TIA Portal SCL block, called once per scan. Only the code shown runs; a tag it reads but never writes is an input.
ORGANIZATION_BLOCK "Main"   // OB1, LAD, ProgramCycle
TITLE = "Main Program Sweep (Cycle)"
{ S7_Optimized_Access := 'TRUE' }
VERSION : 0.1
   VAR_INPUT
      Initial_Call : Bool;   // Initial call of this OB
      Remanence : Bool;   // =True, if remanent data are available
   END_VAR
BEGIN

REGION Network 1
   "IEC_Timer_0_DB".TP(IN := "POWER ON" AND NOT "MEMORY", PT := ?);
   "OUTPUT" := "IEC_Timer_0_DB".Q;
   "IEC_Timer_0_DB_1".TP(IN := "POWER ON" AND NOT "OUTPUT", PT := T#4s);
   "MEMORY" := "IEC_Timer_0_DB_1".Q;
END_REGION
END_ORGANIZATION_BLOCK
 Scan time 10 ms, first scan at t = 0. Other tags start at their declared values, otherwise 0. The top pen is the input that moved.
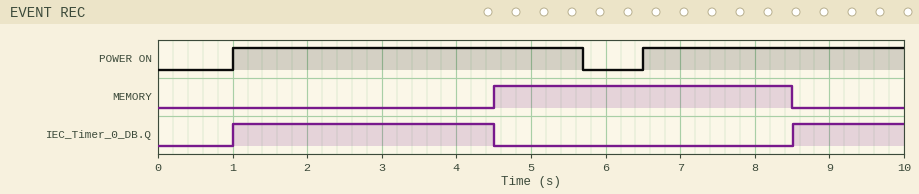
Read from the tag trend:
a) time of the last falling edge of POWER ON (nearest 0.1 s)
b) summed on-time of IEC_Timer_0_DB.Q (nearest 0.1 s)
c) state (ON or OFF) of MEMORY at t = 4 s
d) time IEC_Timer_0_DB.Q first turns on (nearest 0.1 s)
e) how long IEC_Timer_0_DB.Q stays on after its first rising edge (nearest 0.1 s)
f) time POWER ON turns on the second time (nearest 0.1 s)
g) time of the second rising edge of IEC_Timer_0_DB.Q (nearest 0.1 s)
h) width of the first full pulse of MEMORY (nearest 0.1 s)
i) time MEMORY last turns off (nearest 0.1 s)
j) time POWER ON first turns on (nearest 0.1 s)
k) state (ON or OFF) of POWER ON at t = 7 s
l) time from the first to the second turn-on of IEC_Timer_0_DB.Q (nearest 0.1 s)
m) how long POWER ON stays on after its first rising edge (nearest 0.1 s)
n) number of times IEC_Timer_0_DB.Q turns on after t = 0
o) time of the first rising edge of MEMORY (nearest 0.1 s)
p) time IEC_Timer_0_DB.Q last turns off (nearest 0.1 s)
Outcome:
5.7 s
5.0 s
OFF
1.0 s
3.5 s
6.5 s
8.5 s
4.0 s
8.5 s
1.0 s
ON
7.5 s
4.7 s
2
4.5 s
4.5 s
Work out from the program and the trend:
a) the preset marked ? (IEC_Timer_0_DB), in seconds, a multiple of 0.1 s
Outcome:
3.5 s
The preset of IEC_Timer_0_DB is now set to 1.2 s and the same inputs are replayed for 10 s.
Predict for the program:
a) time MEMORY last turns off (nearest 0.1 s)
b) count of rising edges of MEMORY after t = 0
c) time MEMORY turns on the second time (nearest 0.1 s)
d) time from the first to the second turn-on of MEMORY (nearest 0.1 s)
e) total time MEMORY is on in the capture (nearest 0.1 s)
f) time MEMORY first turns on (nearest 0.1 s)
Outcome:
6.2 s
2
7.7 s
5.5 s
6.3 s
2.2 s
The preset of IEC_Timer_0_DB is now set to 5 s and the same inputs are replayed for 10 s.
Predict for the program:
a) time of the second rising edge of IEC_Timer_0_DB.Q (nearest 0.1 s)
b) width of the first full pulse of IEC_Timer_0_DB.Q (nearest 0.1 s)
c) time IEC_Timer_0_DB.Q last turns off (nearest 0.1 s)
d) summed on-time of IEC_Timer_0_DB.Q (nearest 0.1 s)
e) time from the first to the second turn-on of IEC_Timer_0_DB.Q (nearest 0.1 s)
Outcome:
6.5 s
5.0 s
6.0 s
8.5 s
5.5 s
